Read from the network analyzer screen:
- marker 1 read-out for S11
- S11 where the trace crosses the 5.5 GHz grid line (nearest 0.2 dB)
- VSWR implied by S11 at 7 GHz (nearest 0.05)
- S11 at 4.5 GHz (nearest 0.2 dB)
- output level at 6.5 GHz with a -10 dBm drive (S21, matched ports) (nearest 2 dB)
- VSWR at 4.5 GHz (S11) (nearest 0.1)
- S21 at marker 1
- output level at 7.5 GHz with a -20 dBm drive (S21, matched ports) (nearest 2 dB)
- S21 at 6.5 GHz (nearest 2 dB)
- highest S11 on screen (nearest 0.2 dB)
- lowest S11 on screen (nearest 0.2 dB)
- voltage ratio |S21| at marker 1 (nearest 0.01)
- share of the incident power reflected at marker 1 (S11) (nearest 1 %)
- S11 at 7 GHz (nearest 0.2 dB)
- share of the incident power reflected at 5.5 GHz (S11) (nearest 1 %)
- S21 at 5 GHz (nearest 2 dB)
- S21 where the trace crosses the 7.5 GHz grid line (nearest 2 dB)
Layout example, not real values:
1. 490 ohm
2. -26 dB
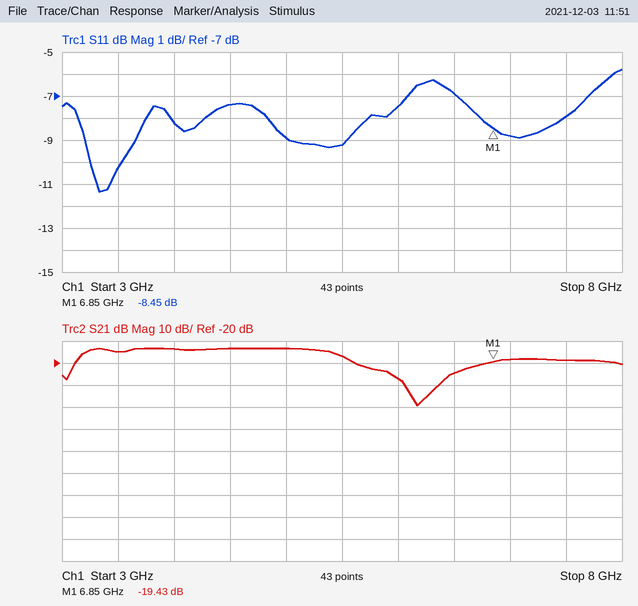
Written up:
1. -8.45 dB
2. -9.2 dB
3. 2.15
4. -7.4 dB
5. -34 dBm
6. 2.5
7. -19.43 dB
8. -38 dBm
9. -24 dB
10. -5.8 dB
11. -11.4 dB
12. 0.11
13. 14 %
14. -8.8 dB
15. 12 %
16. -14 dB
17. -18 dB
